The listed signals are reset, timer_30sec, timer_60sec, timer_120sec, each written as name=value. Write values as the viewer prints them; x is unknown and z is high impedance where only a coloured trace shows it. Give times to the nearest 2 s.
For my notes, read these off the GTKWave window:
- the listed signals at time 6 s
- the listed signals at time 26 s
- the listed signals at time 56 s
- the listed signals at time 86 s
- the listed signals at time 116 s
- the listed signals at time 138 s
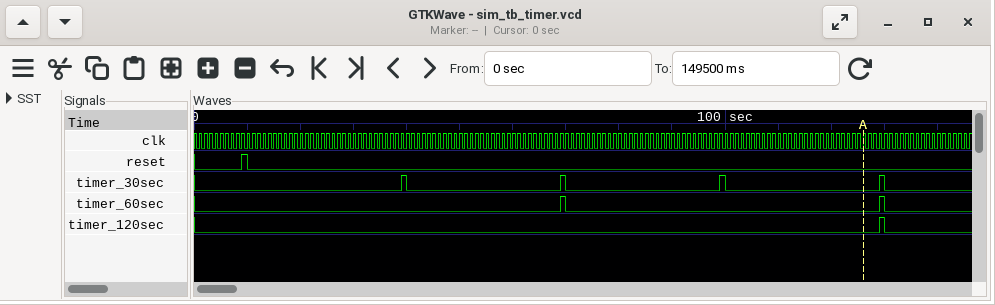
reset=0, timer_30sec=0, timer_60sec=0, timer_120sec=0
reset=0, timer_30sec=0, timer_60sec=0, timer_120sec=0
reset=0, timer_30sec=0, timer_60sec=0, timer_120sec=0
reset=0, timer_30sec=0, timer_60sec=0, timer_120sec=0
reset=0, timer_30sec=0, timer_60sec=0, timer_120sec=0
reset=0, timer_30sec=0, timer_60sec=0, timer_120sec=0
